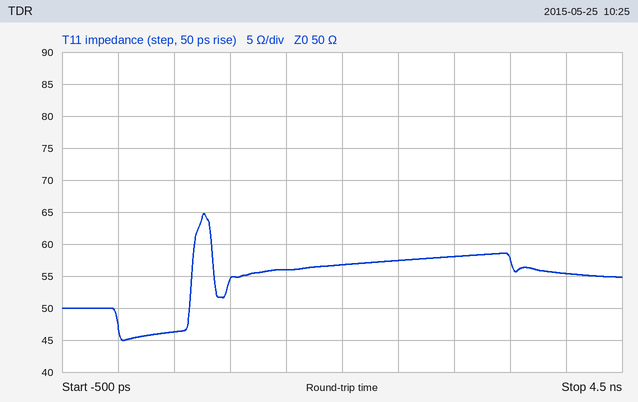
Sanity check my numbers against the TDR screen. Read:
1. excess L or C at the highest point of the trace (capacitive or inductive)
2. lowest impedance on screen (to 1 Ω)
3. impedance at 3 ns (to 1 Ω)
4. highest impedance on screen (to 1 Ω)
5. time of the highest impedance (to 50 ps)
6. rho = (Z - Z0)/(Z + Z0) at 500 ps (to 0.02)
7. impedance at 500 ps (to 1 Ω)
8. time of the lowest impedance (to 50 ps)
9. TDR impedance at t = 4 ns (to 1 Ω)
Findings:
inductive
45 Ω
58 Ω
65 Ω
750 ps
-0.04
46 Ω
50 ps
55 Ω
